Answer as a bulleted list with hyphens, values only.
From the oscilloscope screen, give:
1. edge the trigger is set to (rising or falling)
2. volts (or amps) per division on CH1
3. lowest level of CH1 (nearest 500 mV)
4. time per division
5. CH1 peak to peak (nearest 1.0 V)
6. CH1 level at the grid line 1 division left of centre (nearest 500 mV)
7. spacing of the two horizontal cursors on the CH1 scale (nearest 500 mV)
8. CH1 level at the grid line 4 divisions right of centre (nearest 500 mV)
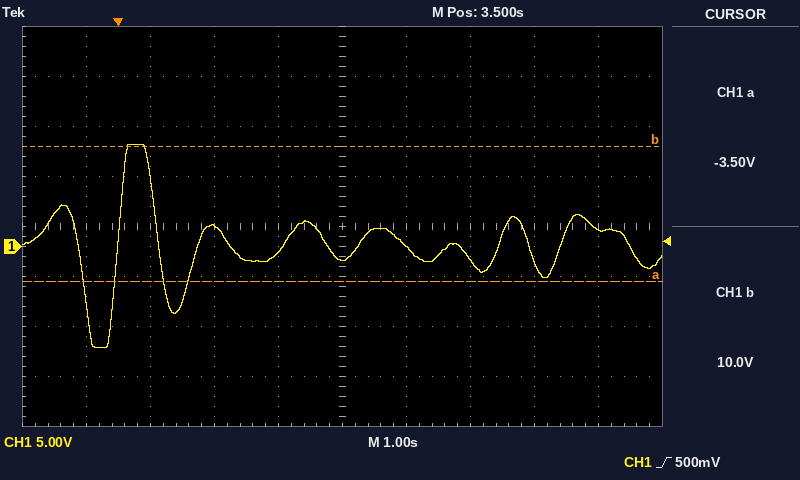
- rising
- 5 V
- -10.0 V
- 1 s
- 20.0 V
- -500 mV
- 13.5 V
- 1.5 V
